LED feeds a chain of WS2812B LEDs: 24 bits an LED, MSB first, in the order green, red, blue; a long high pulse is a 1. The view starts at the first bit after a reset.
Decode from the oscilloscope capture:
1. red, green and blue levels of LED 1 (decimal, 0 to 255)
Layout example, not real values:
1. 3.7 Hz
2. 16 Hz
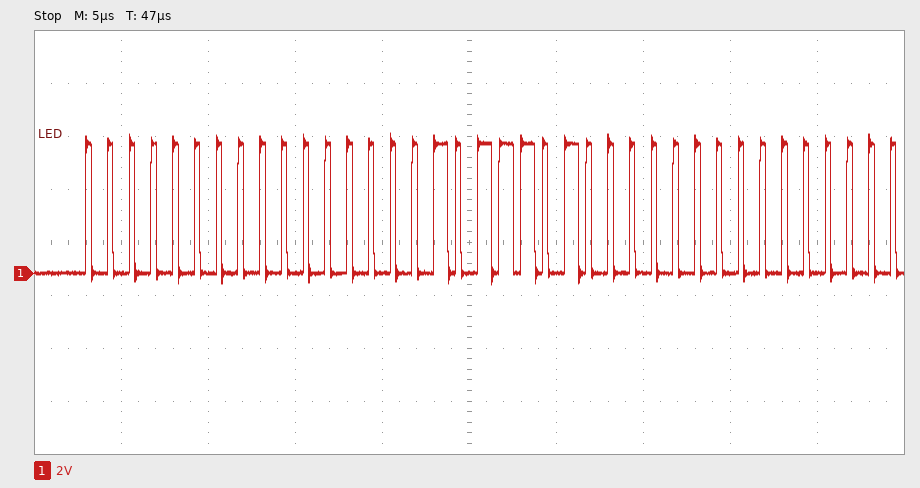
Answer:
1. 0, 0, 186
